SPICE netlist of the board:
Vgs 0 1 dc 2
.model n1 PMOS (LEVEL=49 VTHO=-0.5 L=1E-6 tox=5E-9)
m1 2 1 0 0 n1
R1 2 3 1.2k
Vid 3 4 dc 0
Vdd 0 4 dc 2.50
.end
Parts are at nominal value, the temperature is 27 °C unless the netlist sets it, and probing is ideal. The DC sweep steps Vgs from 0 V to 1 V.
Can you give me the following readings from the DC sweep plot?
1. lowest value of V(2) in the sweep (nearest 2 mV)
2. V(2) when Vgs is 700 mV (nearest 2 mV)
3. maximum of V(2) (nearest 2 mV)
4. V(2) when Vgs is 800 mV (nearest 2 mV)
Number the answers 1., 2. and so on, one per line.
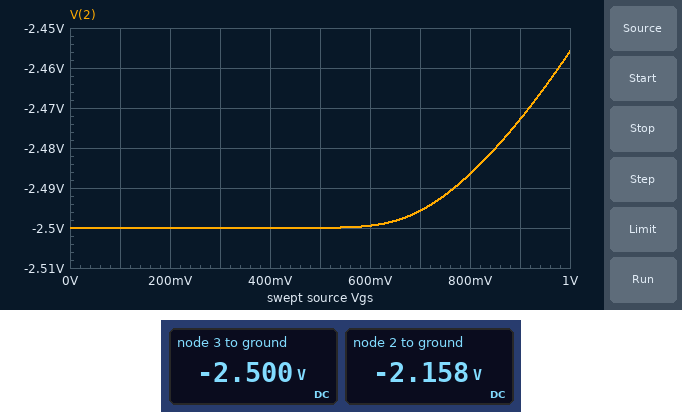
1. -2.500 V
2. -2.496 V
3. -2.456 V
4. -2.486 V
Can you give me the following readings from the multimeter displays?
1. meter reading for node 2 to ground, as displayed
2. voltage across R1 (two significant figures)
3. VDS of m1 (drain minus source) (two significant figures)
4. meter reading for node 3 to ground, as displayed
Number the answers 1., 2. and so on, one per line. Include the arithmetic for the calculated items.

1. -2.158 V
2. -2.158 V - (-2.5 V) = 340 mV
3. -2.158 V = -2.2 V
4. -2.500 V
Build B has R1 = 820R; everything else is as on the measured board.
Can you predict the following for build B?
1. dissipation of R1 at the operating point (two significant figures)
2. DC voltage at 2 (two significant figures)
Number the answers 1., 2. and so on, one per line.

1. 67 µW
2. -2.3 V
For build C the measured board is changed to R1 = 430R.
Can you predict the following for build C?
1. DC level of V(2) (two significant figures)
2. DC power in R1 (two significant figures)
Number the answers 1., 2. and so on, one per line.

1. -2.4 V
2. 35 µW
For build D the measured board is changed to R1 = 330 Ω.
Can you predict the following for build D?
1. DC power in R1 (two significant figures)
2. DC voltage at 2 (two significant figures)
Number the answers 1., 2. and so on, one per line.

1. 27 µW
2. -2.4 V
